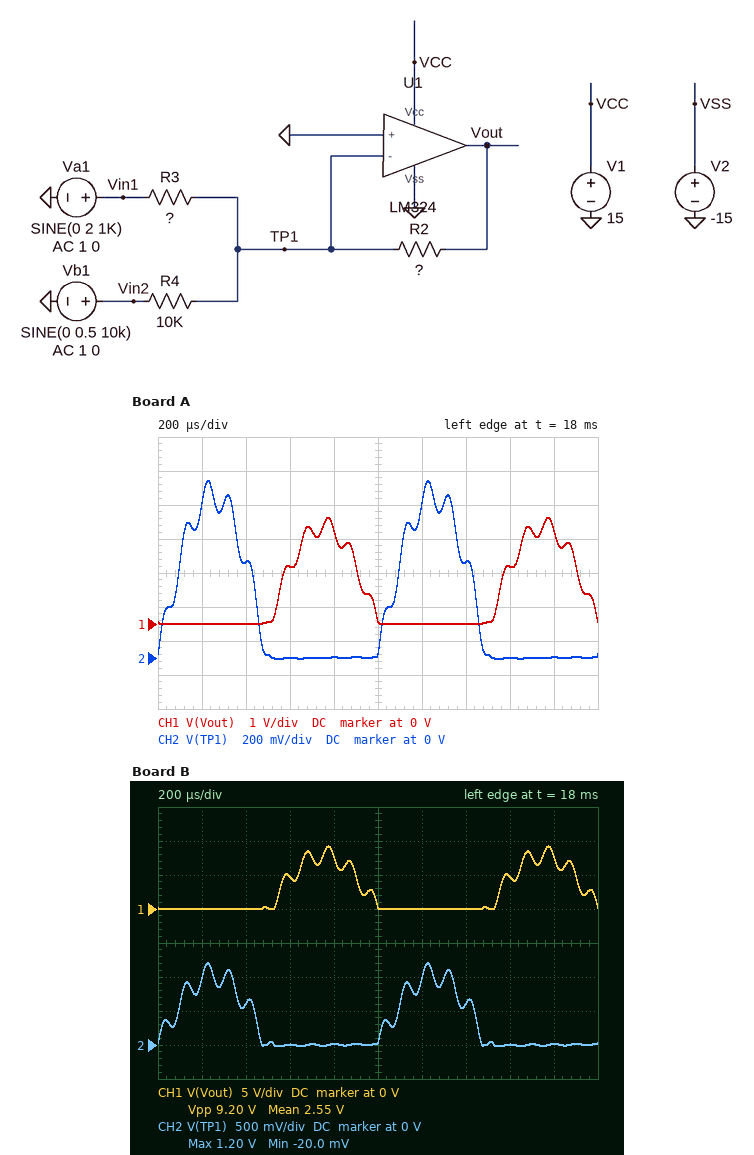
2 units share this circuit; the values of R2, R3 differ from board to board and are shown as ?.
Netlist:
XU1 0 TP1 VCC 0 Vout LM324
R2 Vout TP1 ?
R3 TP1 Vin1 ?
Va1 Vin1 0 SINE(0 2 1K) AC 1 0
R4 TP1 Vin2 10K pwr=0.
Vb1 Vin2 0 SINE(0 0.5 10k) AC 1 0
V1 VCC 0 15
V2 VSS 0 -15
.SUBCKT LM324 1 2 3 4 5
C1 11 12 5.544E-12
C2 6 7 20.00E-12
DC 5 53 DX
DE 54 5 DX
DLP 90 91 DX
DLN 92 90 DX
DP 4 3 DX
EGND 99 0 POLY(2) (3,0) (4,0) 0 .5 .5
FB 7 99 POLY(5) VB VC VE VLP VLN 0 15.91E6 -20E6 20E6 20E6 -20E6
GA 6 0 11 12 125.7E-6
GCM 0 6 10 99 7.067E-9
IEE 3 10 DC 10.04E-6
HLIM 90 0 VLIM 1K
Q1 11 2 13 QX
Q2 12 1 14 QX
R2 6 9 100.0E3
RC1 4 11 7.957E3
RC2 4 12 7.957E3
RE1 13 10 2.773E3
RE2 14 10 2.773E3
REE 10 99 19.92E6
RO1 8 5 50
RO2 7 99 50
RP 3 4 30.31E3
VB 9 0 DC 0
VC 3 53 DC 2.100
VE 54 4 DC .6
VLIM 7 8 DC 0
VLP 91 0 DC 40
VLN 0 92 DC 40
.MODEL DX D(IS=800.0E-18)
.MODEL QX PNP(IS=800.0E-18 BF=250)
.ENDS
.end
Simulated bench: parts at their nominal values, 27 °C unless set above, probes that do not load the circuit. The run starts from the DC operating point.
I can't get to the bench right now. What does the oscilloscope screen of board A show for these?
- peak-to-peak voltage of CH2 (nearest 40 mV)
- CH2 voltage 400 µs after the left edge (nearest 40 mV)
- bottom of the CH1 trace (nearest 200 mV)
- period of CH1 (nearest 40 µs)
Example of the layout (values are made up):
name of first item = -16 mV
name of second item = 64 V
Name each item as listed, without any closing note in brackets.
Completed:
peak-to-peak voltage of CH2 = 1.04 V
CH2 voltage 400 µs after the left edge = 560 mV
bottom of the CH1 trace = 0 V
period of CH1 = 1.00 ms
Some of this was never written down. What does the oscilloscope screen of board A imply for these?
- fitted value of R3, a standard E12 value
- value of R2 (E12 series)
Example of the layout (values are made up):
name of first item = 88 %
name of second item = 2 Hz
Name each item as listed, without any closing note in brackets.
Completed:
fitted value of R3, a standard E12 value = 3.9 kΩ
value of R2 = 5.6 kΩ
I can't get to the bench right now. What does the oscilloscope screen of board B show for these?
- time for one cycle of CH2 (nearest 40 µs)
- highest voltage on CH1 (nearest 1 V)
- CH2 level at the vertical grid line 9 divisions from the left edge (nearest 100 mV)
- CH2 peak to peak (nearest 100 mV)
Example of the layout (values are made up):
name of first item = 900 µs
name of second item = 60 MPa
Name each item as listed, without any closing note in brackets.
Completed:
time for one cycle of CH2 = 1.00 ms
highest voltage on CH1 = 9 V
CH2 level at the vertical grid line 9 divisions from the left edge = 0 V
CH2 peak to peak = 1.2 V
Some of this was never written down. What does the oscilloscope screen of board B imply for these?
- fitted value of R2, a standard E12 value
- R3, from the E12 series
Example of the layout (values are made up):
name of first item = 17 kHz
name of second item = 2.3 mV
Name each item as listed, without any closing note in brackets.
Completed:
fitted value of R2, a standard E12 value = 27 kΩ
R3, from the E12 series = 6.8 kΩ
